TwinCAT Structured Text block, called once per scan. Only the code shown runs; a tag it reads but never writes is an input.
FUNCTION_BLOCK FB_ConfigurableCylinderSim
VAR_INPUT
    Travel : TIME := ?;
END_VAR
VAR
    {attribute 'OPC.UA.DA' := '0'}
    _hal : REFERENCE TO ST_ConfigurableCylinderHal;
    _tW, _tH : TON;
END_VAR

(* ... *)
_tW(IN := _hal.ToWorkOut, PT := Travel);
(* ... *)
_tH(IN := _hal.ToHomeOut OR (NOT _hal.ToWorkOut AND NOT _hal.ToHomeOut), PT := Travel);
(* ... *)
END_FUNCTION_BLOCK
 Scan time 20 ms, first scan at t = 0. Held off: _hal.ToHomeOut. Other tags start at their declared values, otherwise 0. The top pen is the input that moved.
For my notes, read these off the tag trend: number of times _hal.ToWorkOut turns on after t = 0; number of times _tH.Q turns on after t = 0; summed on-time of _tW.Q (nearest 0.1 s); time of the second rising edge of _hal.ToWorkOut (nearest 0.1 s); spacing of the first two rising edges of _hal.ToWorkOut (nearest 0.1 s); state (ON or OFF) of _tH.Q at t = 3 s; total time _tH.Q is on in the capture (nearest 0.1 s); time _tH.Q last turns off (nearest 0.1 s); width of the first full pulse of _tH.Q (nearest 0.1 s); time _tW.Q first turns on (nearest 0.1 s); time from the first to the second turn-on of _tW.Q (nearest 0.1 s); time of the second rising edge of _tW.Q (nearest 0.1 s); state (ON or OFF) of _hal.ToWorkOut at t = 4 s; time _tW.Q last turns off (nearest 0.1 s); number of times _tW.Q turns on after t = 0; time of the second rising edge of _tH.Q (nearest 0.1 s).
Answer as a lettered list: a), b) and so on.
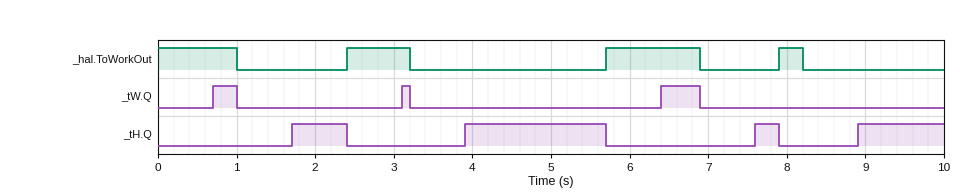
a) 3
b) 4
c) 0.9 s
d) 5.7 s
e) 3.3 s
f) OFF
g) 3.9 s
h) 7.9 s
i) 0.7 s
j) 0.7 s
k) 2.4 s
l) 3.1 s
m) OFF
n) 6.9 s
o) 3
p) 3.9 s
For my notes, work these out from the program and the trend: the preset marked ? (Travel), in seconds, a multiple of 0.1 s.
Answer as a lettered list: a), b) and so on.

a) 0.7 s
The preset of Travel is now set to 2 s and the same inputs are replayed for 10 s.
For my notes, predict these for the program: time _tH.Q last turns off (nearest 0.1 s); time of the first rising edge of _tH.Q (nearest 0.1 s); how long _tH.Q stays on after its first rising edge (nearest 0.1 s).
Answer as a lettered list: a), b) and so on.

a) 5.7 s
b) 5.2 s
c) 0.5 s
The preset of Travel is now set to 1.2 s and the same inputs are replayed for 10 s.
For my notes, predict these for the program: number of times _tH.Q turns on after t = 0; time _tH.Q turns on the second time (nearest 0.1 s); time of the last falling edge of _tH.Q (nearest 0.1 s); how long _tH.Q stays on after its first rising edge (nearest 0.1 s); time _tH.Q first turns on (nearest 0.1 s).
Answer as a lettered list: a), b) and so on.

a) 3
b) 4.4 s
c) 5.7 s
d) 0.2 s
e) 2.2 s
